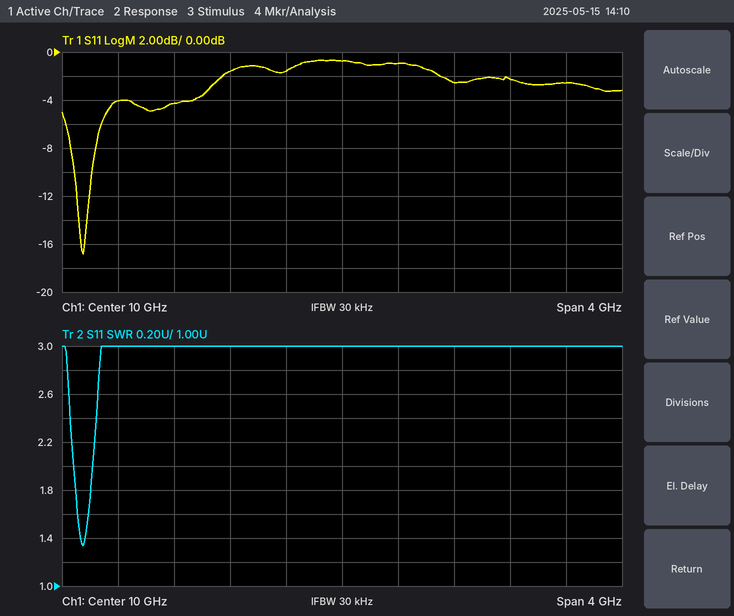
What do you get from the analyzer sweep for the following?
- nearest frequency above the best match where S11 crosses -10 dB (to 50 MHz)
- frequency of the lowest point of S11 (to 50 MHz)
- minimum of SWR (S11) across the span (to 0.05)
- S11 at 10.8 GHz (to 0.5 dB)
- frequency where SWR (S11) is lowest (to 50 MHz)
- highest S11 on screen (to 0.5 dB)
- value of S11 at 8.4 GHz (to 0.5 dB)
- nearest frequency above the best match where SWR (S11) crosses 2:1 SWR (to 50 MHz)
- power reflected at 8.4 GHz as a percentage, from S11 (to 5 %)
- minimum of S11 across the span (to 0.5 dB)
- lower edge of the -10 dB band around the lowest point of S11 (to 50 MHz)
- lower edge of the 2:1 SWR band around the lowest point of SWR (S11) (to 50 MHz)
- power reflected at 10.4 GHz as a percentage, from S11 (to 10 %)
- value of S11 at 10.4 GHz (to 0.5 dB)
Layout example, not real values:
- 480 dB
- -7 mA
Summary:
- 8.20 GHz
- 8.15 GHz
- 1.35
- -2.5 dB
- 8.15 GHz
- -0.5 dB
- -4.0 dB
- 8.20 GHz
- 40 %
- -17.0 dB
- 8.10 GHz
- 8.10 GHz
- 80 %
- -1.0 dB
